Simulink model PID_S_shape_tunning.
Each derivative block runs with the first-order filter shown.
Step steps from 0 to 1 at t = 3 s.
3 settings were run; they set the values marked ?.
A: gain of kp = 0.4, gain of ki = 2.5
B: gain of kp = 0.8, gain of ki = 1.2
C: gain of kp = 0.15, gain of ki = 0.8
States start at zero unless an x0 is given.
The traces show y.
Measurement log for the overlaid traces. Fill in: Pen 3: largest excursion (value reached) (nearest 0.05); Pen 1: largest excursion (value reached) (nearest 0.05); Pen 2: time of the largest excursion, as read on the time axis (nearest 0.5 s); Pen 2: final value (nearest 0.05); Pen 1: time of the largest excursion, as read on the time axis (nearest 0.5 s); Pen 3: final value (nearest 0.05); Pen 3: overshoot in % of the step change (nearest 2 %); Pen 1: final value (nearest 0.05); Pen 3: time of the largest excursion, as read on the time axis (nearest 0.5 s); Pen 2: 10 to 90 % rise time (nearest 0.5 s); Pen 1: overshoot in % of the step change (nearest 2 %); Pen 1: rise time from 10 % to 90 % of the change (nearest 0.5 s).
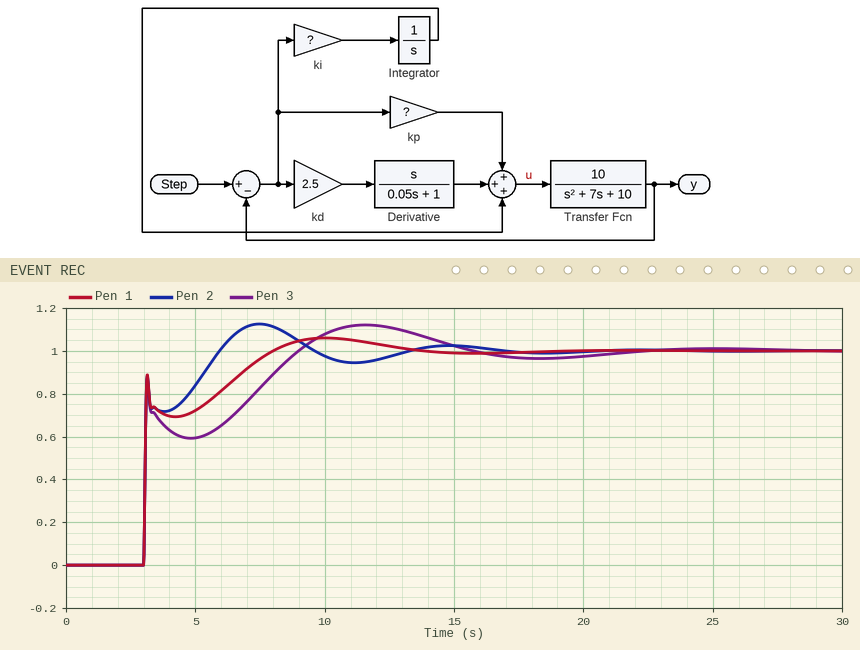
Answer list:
1.10
1.05
7.5 s
1.00
10.0 s
1.00
12 %
1.00
11.5 s
2.5 s
6 %
4.0 s
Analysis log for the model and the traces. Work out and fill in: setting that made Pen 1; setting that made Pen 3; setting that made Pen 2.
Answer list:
B
C
A
